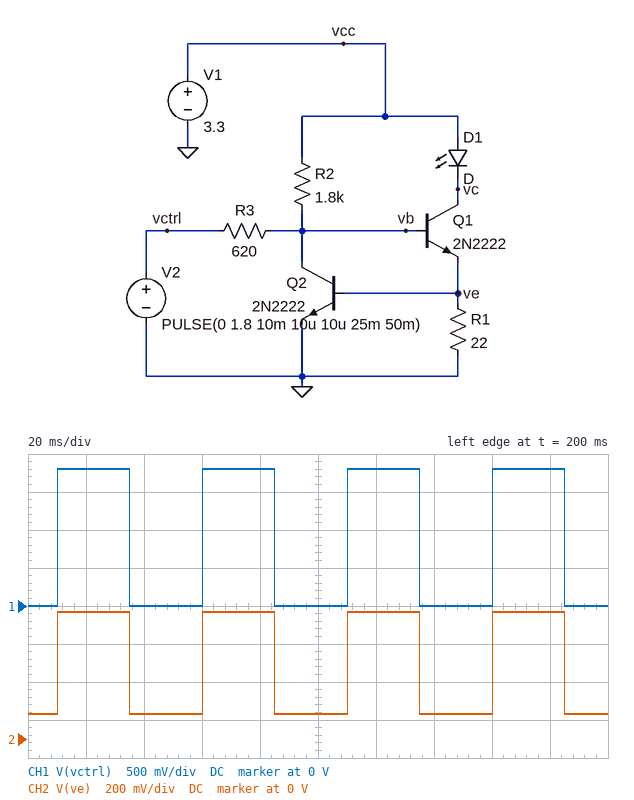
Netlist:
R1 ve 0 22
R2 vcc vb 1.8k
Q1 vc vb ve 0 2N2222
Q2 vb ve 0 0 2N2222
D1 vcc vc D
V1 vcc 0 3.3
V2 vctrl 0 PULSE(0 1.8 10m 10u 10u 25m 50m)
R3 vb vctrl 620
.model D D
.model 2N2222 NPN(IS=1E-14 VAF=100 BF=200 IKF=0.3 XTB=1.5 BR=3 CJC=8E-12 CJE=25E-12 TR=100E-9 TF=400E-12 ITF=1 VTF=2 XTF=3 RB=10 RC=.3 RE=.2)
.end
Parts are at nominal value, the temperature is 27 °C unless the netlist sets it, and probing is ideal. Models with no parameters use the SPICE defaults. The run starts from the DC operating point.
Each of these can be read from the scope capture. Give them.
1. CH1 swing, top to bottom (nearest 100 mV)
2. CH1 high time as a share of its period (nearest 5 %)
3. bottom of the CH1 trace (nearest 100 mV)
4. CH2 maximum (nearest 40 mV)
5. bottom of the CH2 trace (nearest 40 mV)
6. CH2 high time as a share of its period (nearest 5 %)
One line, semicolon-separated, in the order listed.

1.8 V; 50 %; 0 V; 680 mV; 120 mV; 50 %
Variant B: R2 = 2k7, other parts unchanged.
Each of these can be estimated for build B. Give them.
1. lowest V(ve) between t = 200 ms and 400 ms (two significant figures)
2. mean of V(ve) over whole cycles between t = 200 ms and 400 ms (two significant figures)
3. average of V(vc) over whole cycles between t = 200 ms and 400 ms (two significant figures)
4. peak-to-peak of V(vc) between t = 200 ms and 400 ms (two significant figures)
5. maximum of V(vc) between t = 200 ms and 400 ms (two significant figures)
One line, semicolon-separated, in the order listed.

4.2 mV; 330 mV; 2.6 V; 130 mV; 2.7 V
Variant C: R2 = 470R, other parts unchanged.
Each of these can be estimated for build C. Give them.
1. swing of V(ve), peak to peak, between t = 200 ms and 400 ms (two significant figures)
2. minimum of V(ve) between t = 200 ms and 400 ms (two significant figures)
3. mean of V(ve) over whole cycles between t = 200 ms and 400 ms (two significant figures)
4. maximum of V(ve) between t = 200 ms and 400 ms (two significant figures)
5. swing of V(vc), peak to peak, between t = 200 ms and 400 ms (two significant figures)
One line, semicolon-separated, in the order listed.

28 mV; 670 mV; 680 mV; 690 mV; 1.1 mV
